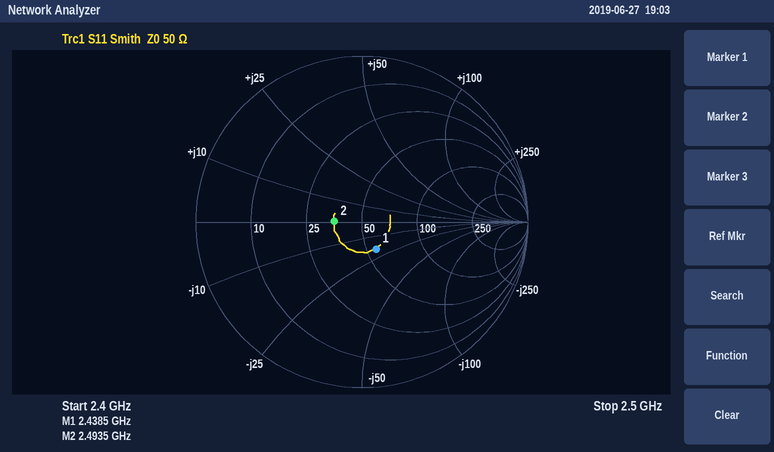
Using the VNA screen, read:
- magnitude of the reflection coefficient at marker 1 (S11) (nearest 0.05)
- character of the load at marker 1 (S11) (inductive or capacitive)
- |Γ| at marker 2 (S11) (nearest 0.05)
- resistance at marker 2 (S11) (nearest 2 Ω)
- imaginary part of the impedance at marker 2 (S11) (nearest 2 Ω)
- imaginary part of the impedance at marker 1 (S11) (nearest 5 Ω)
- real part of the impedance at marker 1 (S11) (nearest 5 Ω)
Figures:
0.20
capacitive
0.15
36 Ω
0 Ω
-20 Ω
55 Ω
